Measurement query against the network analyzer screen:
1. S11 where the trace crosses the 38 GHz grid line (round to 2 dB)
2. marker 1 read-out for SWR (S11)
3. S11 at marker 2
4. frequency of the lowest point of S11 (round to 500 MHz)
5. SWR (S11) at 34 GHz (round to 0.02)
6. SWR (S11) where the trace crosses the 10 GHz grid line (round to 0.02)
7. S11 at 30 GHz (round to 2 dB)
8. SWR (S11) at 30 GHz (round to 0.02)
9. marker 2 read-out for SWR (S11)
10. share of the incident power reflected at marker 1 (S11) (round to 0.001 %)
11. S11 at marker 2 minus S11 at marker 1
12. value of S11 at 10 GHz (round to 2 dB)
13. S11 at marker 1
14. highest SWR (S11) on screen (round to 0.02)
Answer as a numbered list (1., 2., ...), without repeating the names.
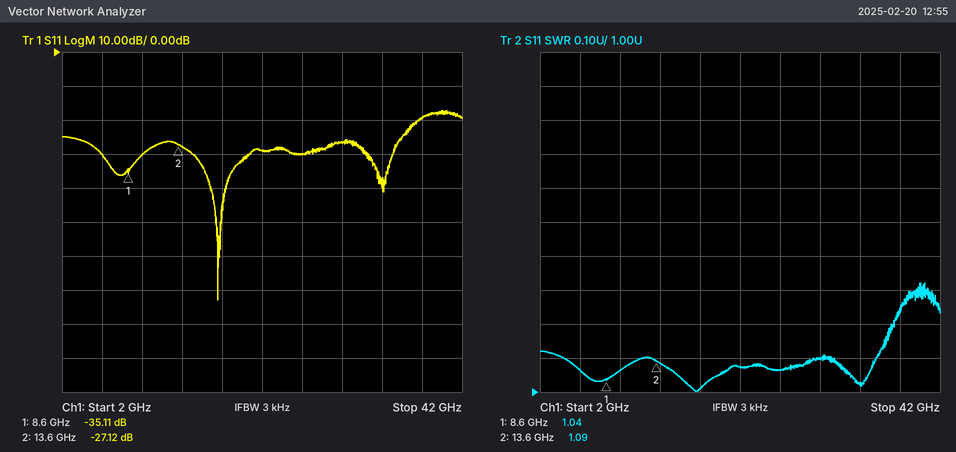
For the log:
1. -20 dB
2. 1.04
3. -27.12 dB
4. 17.5 GHz
5. 1.02
6. 1.06
7. -26 dB
8. 1.10
9. 1.09
10. 0.031 %
11. 7.99 dB
12. -30 dB
13. -35.11 dB
14. 1.32
